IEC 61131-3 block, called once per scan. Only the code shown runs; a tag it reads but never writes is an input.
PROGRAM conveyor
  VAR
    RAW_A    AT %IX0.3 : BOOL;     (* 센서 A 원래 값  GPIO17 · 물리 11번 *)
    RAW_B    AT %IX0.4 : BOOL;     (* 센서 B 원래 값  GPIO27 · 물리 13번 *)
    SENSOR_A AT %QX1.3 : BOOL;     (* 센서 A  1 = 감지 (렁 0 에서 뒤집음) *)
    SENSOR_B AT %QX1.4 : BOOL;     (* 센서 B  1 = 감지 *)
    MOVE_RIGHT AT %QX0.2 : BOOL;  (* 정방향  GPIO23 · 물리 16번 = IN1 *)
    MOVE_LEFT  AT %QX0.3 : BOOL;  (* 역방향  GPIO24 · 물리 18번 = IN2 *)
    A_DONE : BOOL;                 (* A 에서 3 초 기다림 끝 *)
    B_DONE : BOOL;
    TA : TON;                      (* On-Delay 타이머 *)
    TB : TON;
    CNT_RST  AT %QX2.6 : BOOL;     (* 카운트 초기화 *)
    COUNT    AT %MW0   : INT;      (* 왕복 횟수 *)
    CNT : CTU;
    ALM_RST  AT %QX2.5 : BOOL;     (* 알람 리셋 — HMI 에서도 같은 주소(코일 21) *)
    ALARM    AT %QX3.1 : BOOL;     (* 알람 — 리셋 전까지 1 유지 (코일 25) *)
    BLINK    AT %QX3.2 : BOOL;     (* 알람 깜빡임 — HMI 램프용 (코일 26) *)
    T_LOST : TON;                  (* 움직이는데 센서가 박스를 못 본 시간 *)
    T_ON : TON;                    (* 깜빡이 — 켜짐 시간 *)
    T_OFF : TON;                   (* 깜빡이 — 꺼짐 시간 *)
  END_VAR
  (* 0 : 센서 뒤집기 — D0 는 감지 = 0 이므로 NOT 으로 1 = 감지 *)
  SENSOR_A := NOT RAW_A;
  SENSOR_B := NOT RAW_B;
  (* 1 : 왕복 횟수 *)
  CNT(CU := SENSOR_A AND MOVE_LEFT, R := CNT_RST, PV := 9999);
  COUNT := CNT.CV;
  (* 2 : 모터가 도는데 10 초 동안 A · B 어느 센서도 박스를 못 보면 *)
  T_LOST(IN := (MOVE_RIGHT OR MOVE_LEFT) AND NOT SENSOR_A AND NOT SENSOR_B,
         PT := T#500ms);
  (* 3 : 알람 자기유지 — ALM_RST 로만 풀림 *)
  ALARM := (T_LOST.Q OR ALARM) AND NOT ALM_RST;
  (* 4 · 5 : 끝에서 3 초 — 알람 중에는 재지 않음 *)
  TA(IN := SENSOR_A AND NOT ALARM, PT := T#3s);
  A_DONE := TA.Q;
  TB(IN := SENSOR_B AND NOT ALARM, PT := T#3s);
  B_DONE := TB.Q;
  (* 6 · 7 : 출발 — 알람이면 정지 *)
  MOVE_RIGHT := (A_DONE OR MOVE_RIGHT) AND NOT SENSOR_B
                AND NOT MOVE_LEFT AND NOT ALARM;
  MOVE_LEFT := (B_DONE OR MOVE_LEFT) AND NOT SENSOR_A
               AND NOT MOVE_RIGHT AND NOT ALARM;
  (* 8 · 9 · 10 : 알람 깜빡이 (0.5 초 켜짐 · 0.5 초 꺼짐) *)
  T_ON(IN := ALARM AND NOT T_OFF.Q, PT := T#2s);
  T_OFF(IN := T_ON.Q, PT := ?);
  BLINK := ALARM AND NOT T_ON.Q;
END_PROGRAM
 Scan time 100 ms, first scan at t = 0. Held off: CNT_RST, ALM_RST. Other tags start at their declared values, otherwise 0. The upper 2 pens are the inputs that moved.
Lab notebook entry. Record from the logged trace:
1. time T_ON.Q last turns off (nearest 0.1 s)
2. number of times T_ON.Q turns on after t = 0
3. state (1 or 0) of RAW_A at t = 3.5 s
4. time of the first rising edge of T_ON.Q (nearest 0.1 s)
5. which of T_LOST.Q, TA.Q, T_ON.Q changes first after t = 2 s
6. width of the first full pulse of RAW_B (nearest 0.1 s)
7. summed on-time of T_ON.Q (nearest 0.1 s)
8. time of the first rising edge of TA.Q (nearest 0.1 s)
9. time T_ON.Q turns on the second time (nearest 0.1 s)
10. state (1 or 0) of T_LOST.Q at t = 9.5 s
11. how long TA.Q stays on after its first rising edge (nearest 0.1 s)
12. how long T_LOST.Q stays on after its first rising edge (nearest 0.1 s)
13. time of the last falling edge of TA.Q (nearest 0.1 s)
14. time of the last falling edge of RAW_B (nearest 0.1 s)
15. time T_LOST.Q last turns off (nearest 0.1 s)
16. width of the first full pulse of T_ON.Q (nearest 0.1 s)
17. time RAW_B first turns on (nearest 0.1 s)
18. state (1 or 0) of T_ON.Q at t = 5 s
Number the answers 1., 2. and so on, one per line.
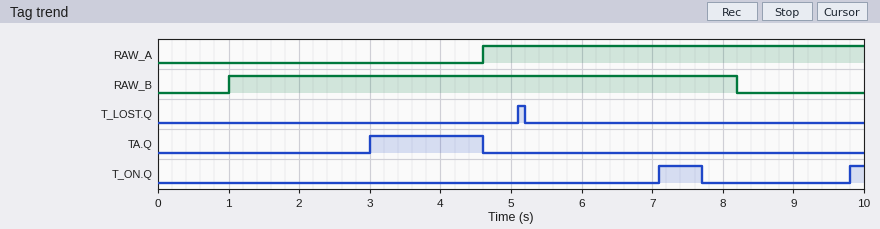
1. 7.7 s
2. 2
3. 0
4. 7.1 s
5. TA.Q
6. 7.2 s
7. 0.8 s
8. 3.0 s
9. 9.8 s
10. 0
11. 1.6 s
12. 0.1 s
13. 4.6 s
14. 8.2 s
15. 5.2 s
16. 0.6 s
17. 1.0 s
18. 0
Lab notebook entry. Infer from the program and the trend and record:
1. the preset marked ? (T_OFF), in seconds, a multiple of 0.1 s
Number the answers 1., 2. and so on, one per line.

1. 0.5 s
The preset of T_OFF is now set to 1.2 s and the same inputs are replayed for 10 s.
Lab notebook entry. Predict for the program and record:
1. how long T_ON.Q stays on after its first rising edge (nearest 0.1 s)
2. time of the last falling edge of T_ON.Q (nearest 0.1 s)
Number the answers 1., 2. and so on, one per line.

1. 1.3 s
2. 8.4 s
